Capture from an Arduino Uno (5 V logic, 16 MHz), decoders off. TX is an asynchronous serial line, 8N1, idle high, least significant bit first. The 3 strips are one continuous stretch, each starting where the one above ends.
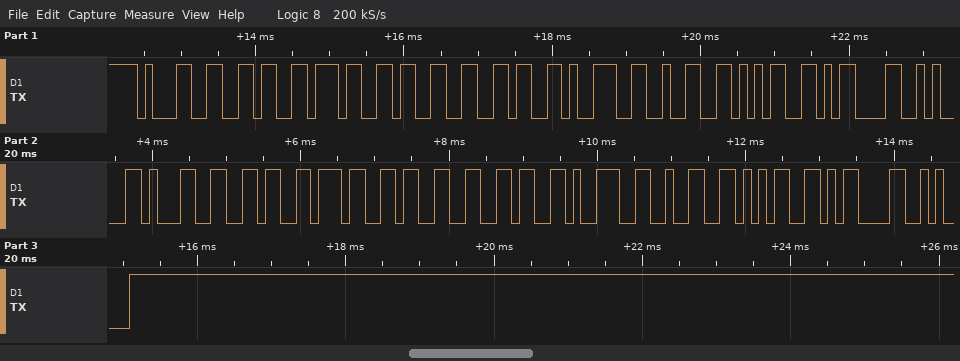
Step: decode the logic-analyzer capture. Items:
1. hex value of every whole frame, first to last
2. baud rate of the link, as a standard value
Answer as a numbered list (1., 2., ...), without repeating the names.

1. 31 36 37 33 36 39 32 35 0D 0A 31 36 37 33 36 39 32 35 0D 0A
2. 9600 baud
